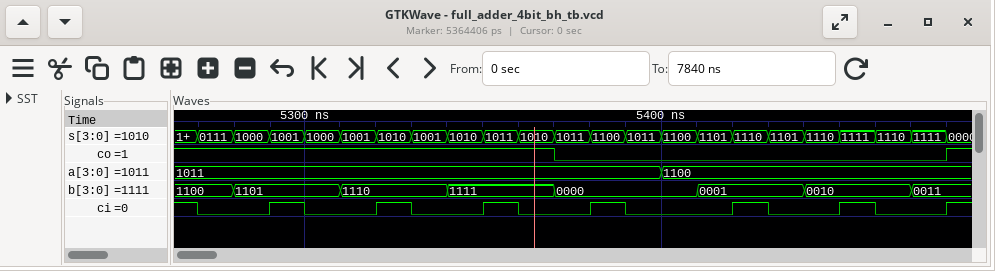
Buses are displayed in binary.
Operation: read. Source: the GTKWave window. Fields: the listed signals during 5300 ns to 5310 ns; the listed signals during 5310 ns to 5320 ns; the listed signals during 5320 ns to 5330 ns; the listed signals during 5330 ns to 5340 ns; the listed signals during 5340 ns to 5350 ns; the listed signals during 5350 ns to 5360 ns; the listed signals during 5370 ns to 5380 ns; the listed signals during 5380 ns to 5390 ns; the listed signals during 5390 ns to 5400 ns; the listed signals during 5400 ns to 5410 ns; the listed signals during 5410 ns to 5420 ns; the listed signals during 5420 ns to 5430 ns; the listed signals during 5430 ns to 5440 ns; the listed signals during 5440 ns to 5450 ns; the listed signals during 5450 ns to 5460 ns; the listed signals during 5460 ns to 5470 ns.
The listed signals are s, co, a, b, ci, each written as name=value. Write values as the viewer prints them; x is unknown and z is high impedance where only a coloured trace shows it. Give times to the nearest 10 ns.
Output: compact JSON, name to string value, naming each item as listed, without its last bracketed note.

{"the listed signals during 5300 ns to 5310 ns": "s=1000, co=1, a=1011, b=1101, ci=0", "the listed signals during 5310 ns to 5320 ns": "s=1001, co=1, a=1011, b=1110, ci=0", "the listed signals during 5320 ns to 5330 ns": "s=1010, co=1, a=1011, b=1110, ci=1", "the listed signals during 5330 ns to 5340 ns": "s=1001, co=1, a=1011, b=1110, ci=0", "the listed signals during 5340 ns to 5350 ns": "s=1010, co=1, a=1011, b=1111, ci=0", "the listed signals during 5350 ns to 5360 ns": "s=1011, co=1, a=1011, b=1111, ci=1", "the listed signals during 5370 ns to 5380 ns": "s=1011, co=0, a=1011, b=0000, ci=0", "the listed signals during 5380 ns to 5390 ns": "s=1100, co=0, a=1011, b=0000, ci=1", "the listed signals during 5390 ns to 5400 ns": "s=1011, co=0, a=1011, b=0000, ci=0", "the listed signals during 5400 ns to 5410 ns": "s=1100, co=0, a=1100, b=0000, ci=0", "the listed signals during 5410 ns to 5420 ns": "s=1101, co=0, a=1100, b=0001, ci=0", "the listed signals during 5420 ns to 5430 ns": "s=1110, co=0, a=1100, b=0001, ci=1", "the listed signals during 5430 ns to 5440 ns": "s=1101, co=0, a=1100, b=0001, ci=0", "the listed signals during 5440 ns to 5450 ns": "s=1110, co=0, a=1100, b=0010, ci=0", "the listed signals during 5450 ns to 5460 ns": "s=1111, co=0, a=1100, b=0010, ci=1", "the listed signals during 5460 ns to 5470 ns": "s=1110, co=0, a=1100, b=0010, ci=0"}
